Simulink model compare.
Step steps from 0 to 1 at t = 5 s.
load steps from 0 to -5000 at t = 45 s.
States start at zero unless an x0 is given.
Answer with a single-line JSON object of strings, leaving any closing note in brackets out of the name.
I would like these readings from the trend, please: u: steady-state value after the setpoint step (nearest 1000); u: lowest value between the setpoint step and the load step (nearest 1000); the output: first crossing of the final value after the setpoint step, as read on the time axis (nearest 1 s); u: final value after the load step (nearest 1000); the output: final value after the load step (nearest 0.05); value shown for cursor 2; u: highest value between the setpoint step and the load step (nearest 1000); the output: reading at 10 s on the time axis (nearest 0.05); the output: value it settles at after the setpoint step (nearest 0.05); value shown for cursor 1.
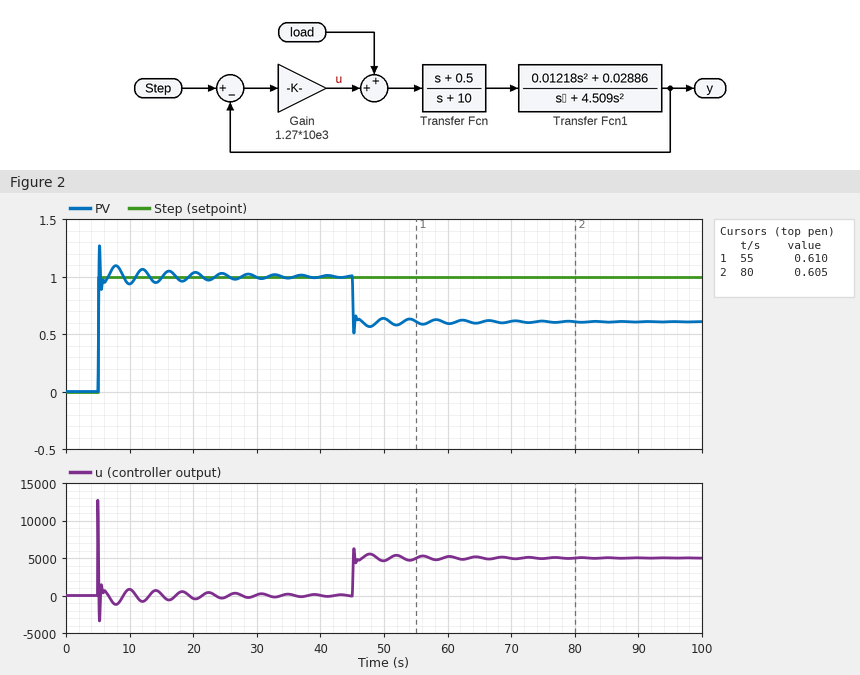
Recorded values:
{"u: steady-state value after the setpoint step": "0", "u: lowest value between the setpoint step and the load step": "-3000", "the output: first crossing of the final value after the setpoint step, as read on the time axis": "5 s", "u: final value after the load step": "5000", "the output: final value after the load step": "0.60", "value shown for cursor 2": "0.605", "u: highest value between the setpoint step and the load step": "13000", "the output: reading at 10 s on the time axis": "0.95", "the output: value it settles at after the setpoint step": "1.00", "value shown for cursor 1": "0.610"}
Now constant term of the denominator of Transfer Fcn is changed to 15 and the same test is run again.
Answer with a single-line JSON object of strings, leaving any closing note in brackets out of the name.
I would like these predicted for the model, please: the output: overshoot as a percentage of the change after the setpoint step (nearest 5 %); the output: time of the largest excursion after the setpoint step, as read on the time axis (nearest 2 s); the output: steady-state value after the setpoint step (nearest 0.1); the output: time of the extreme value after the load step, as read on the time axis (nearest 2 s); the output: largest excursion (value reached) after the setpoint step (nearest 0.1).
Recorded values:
{"the output: overshoot as a percentage of the change after the setpoint step": "15 %", "the output: time of the largest excursion after the setpoint step, as read on the time axis": "8 s", "the output: steady-state value after the setpoint step": "1.0", "the output: time of the extreme value after the load step, as read on the time axis": "48 s", "the output: largest excursion (value reached) after the setpoint step": "1.1"}
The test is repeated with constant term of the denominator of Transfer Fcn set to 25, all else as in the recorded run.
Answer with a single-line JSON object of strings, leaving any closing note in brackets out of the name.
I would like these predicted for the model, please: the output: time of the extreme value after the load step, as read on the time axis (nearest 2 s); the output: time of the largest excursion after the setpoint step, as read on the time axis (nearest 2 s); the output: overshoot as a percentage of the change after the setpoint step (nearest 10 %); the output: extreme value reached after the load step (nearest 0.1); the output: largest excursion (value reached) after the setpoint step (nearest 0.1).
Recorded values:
{"the output: time of the extreme value after the load step, as read on the time axis": "48 s", "the output: time of the largest excursion after the setpoint step, as read on the time axis": "8 s", "the output: overshoot as a percentage of the change after the setpoint step": "20 %", "the output: extreme value reached after the load step": "0.5", "the output: largest excursion (value reached) after the setpoint step": "1.2"}
